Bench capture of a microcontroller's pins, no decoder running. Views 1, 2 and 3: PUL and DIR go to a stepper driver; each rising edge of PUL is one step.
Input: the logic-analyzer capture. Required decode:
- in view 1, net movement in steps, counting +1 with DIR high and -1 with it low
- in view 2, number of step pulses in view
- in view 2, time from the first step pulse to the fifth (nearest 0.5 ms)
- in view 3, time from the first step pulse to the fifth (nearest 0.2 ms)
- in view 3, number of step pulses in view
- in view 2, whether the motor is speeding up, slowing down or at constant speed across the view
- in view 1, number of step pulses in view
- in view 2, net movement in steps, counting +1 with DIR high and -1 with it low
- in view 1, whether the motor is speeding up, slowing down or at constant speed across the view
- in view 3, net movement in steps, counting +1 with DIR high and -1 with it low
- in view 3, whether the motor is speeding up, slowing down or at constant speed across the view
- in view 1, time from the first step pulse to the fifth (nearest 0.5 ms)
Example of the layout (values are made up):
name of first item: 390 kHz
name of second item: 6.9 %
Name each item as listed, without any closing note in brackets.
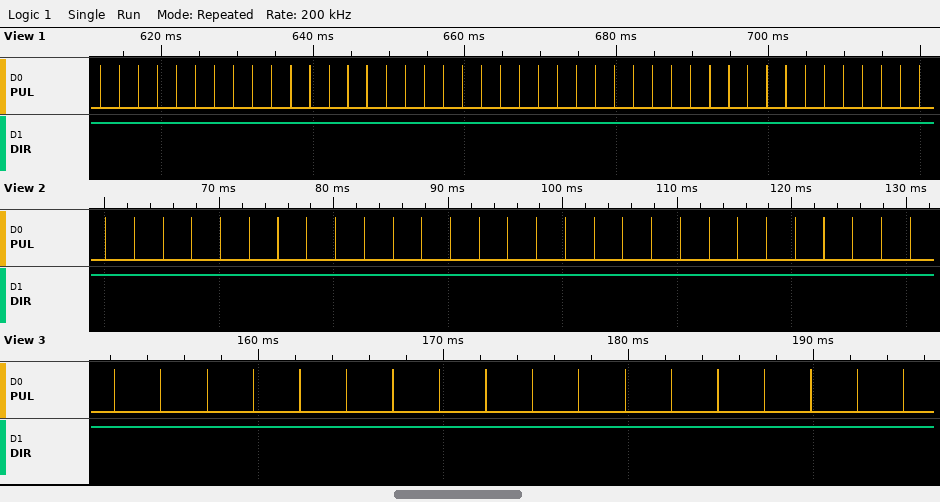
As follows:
in view 1, net movement in steps, counting +1 with DIR high and -1 with it low: +44
in view 2, number of step pulses in view: 29
in view 2, time from the first step pulse to the fifth: 10.0 ms
in view 3, time from the first step pulse to the fifth: 10.0 ms
in view 3, number of step pulses in view: 18
in view 2, whether the motor is speeding up, slowing down or at constant speed across the view: constant speed
in view 1, number of step pulses in view: 44
in view 2, net movement in steps, counting +1 with DIR high and -1 with it low: +29
in view 1, whether the motor is speeding up, slowing down or at constant speed across the view: constant speed
in view 3, net movement in steps, counting +1 with DIR high and -1 with it low: +18
in view 3, whether the motor is speeding up, slowing down or at constant speed across the view: constant speed
in view 1, time from the first step pulse to the fifth: 10.0 ms
